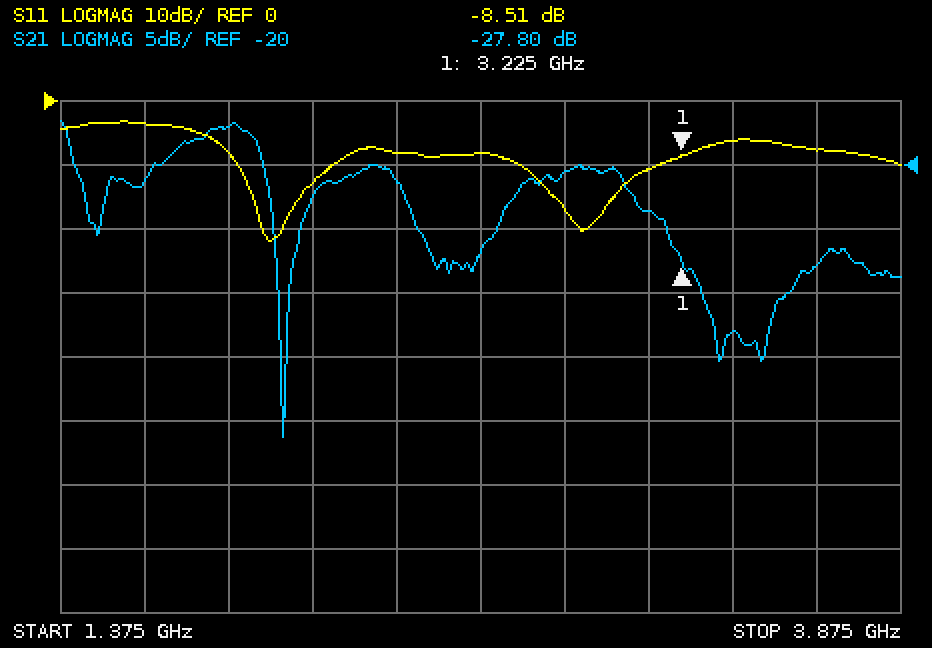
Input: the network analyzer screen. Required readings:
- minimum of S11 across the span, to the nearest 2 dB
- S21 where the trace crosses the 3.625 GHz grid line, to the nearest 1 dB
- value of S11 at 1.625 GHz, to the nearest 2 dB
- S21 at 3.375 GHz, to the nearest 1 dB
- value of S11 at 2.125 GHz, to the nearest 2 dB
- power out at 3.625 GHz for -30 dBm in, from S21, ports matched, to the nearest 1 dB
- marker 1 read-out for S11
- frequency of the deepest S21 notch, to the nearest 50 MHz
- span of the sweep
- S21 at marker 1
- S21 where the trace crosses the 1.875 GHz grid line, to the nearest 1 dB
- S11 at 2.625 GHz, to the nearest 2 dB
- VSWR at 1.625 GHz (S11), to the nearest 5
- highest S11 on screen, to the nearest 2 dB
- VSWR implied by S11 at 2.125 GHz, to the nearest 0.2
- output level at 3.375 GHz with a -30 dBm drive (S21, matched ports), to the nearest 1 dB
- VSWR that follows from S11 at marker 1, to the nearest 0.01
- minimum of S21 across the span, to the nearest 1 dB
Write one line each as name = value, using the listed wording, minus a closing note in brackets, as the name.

minimum of S11 across the span, to the nearest 2 dB = -22 dB
S21 where the trace crosses the 3.625 GHz grid line, to the nearest 1 dB = -28 dB
value of S11 at 1.625 GHz, to the nearest 2 dB = -4 dB
S21 at 3.375 GHz, to the nearest 1 dB = -33 dB
value of S11 at 2.125 GHz, to the nearest 2 dB = -12 dB
power out at 3.625 GHz for -30 dBm in, from S21, ports matched, to the nearest 1 dB = -58 dBm
marker 1 read-out for S11 = -8.51 dB
frequency of the deepest S21 notch, to the nearest 50 MHz = 2.05 GHz
span of the sweep = 2.5 GHz
S21 at marker 1 = -27.80 dB
S21 where the trace crosses the 1.875 GHz grid line, to the nearest 1 dB = -17 dB
S11 at 2.625 GHz, to the nearest 2 dB = -8 dB
VSWR at 1.625 GHz (S11), to the nearest 5 = 5
highest S11 on screen, to the nearest 2 dB = -4 dB
VSWR implied by S11 at 2.125 GHz, to the nearest 0.2 = 1.6
output level at 3.375 GHz with a -30 dBm drive (S21, matched ports), to the nearest 1 dB = -63 dBm
VSWR that follows from S11 at marker 1, to the nearest 0.01 = 2.20
minimum of S21 across the span, to the nearest 1 dB = -41 dB
